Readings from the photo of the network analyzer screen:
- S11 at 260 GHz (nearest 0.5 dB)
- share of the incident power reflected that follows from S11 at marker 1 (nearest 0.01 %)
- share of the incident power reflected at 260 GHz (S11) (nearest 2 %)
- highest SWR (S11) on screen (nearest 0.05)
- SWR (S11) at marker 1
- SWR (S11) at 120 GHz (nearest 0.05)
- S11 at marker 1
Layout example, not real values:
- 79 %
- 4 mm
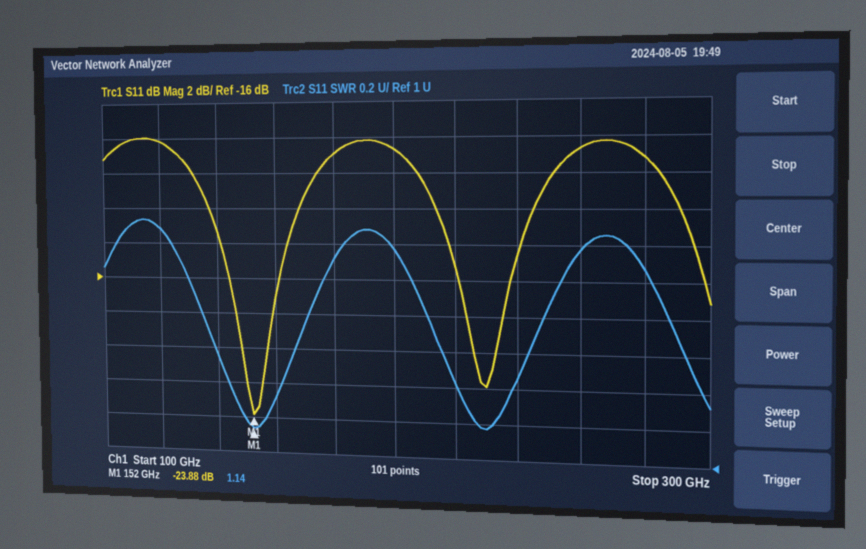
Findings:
- -8.5 dB
- 0.41 %
- 14 %
- 2.35
- 1.14
- 2.30
- -23.88 dB
